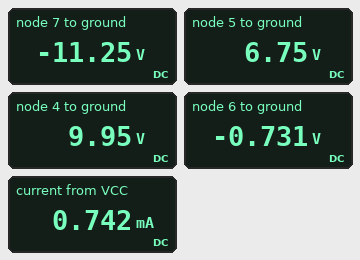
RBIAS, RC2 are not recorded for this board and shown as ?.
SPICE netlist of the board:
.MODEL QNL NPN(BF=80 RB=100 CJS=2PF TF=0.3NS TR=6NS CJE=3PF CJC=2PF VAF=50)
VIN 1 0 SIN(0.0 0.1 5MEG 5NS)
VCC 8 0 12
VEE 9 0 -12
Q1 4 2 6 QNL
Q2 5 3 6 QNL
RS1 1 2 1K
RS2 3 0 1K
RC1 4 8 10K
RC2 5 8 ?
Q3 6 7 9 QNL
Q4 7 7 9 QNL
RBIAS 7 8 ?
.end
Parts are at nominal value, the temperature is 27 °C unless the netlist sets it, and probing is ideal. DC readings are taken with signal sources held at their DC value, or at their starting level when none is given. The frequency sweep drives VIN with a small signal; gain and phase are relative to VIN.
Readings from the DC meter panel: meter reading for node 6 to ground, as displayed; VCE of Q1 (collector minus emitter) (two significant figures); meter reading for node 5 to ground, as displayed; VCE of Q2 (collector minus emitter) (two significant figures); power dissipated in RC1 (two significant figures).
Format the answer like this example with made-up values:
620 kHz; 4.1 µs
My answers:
-0.731 V; 11 V; 6.75 V; 7.5 V; 420 µW
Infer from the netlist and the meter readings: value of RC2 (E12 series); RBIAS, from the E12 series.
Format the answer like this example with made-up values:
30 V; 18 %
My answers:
27 kΩ; 68 kΩ
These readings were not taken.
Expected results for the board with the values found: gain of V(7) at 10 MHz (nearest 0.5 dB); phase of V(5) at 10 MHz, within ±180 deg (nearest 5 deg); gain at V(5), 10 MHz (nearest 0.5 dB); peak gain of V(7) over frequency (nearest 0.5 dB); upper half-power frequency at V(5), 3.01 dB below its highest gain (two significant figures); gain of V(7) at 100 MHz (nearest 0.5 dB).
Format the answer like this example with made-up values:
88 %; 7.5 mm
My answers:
-53.5 dB; -105 deg; 15.0 dB; -41.0 dB; 810 kHz; -41.0 dB
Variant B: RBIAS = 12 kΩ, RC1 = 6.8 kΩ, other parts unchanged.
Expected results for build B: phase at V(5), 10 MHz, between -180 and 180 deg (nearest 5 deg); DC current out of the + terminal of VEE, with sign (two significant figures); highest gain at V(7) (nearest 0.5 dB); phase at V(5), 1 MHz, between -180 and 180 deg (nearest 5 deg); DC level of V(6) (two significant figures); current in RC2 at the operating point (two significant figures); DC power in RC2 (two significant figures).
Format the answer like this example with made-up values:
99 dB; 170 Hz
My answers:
-35 deg; -4.2 mA; -57.0 dB; -5 deg; -810 mV; 470 µA; 6.0 mW
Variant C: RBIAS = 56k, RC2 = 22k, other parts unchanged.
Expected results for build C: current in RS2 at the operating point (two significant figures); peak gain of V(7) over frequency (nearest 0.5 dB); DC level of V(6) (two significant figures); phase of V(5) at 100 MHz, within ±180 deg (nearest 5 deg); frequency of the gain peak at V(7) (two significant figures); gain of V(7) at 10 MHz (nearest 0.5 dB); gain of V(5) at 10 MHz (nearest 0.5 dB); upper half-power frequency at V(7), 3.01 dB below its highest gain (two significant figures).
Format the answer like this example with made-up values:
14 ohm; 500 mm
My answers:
2.6 µA; -42.5 dB; -740 mV; -155 deg; 87 MHz; -55.5 dB; 15.5 dB; 200 MHz
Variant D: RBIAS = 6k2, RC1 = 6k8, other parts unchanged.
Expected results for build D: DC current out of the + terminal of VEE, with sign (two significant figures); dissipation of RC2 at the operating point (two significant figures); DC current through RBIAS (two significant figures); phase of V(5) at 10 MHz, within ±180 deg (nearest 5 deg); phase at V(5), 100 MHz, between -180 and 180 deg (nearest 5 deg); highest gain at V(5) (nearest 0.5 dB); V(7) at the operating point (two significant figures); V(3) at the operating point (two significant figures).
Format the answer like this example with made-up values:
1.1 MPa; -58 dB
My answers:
-8.1 mA; 7.0 mW; 3.7 mA; -25 deg; -50 deg; -7.0 dB; -11 V; -910 mV
